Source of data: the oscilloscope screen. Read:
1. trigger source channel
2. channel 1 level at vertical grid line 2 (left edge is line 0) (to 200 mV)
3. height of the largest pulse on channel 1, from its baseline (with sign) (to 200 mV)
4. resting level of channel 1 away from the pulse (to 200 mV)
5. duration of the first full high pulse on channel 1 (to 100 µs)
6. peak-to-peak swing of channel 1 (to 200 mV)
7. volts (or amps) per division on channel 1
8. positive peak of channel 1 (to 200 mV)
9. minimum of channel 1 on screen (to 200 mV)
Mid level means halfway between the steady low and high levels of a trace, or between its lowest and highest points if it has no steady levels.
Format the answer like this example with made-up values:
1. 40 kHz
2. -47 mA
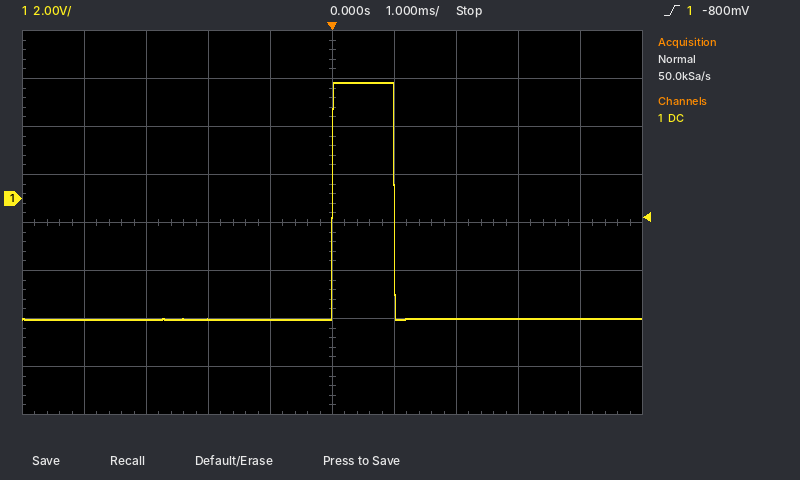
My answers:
1. channel 1
2. -5.0 V
3. +9.8 V
4. -5.0 V
5. 1.0 ms
6. 9.8 V
7. 2 V
8. 4.8 V
9. -5.0 V
